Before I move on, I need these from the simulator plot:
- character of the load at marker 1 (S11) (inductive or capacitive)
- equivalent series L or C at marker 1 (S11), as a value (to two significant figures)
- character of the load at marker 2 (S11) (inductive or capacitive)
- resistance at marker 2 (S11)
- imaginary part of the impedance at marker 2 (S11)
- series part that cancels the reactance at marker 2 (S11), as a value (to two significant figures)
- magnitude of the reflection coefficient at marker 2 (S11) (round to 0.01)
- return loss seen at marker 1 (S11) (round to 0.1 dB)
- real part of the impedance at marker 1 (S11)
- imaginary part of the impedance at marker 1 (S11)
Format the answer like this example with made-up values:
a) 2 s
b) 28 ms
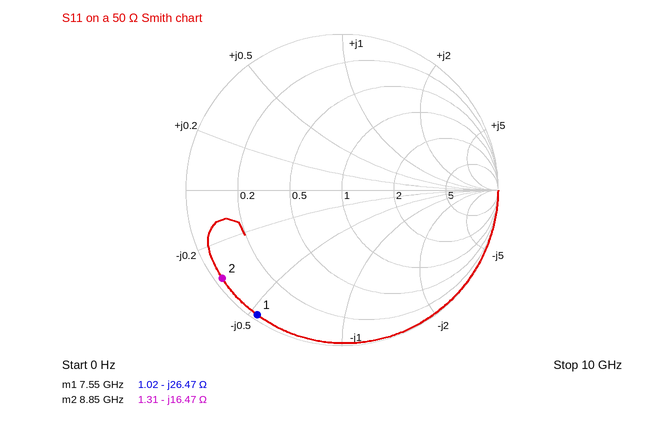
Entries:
a) capacitive
b) 800 fF
c) capacitive
d) 1.31 Ω
e) -16.47 Ω
f) 300 pH
g) 0.95
h) 0.3 dB
i) 1.02 Ω
j) -26.47 Ω
